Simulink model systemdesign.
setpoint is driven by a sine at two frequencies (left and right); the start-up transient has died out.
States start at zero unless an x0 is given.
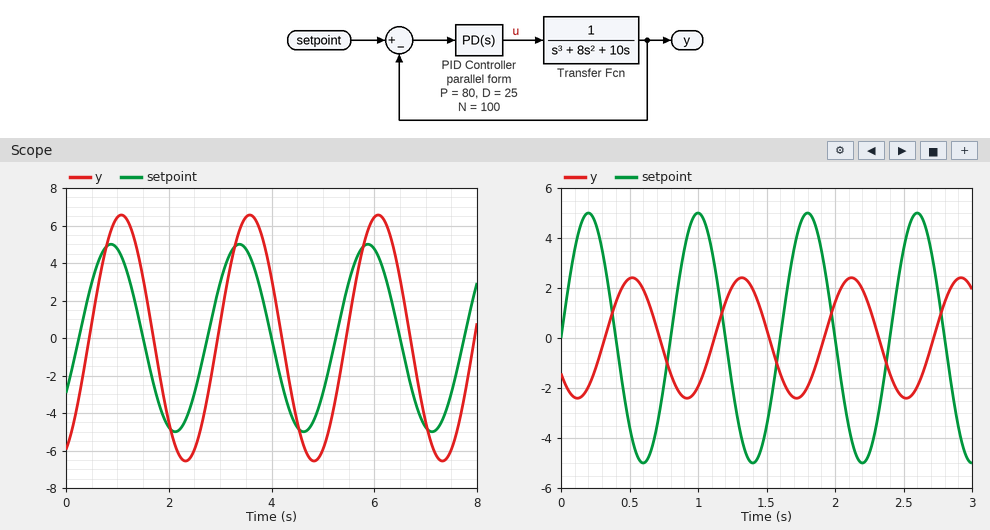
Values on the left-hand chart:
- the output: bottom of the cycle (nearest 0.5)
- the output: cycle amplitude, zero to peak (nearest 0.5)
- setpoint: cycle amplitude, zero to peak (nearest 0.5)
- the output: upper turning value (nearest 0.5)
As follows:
-6.5
6.5
5.0
6.5
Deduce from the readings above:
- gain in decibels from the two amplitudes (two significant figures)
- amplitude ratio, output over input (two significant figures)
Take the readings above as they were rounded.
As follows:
2.3 dB
1.3
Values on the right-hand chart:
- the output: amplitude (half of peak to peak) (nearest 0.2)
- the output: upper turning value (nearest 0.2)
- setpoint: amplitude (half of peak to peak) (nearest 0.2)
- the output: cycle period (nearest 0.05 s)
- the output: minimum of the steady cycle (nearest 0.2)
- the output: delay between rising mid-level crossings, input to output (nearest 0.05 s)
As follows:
2.4
2.4
5.0
0.80 s
-2.4
0.30 s
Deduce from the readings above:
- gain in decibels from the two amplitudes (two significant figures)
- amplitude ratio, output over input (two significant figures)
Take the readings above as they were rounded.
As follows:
-6.4 dB
0.48
